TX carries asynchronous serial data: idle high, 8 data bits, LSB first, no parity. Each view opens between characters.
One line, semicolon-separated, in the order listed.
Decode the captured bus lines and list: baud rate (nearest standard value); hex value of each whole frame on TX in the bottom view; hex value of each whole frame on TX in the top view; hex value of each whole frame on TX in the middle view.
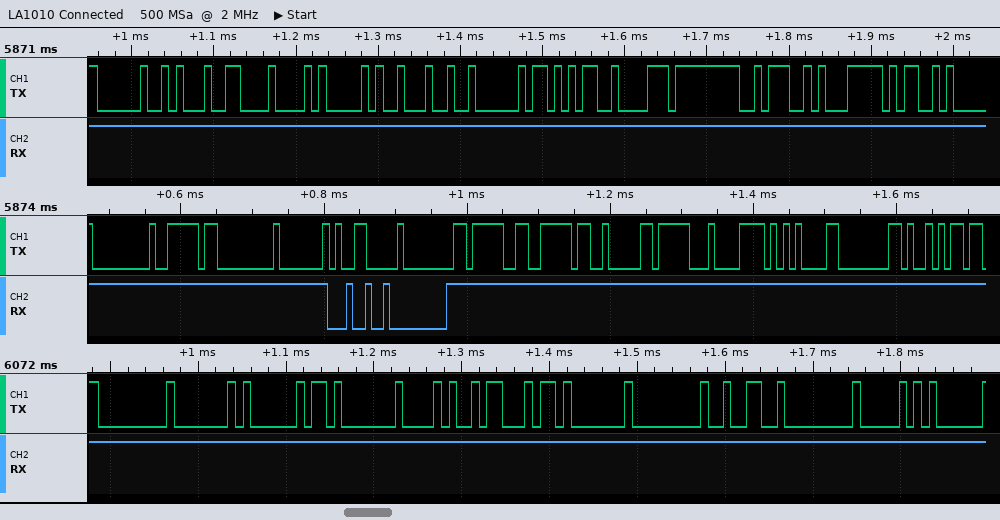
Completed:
115200 baud; 00, 40, A0, 01, 28, A3, 01, 00, 32, 00, 50; 20, 91, 08, 41, 22, 02, AB, C2, FF, 3A, F1, 4D; 00, BE, 00, 40, 06, 80, 9F, BE, 82, 1F, 78, 85, 80, A9
